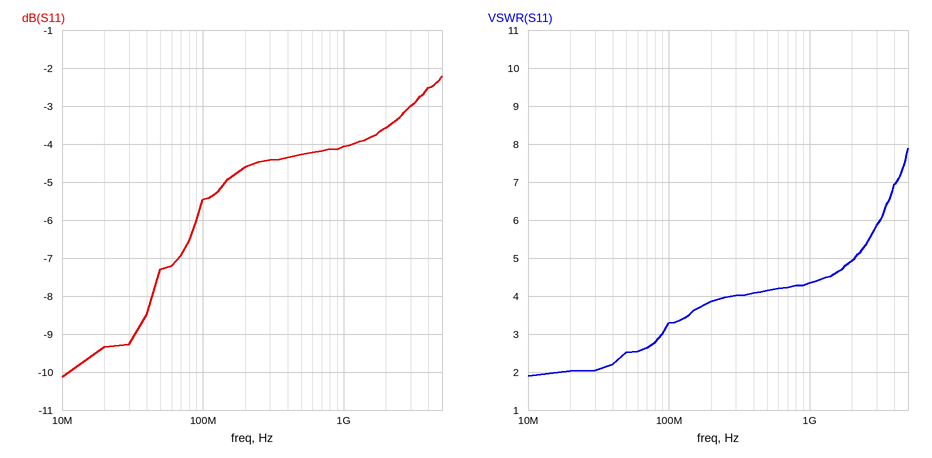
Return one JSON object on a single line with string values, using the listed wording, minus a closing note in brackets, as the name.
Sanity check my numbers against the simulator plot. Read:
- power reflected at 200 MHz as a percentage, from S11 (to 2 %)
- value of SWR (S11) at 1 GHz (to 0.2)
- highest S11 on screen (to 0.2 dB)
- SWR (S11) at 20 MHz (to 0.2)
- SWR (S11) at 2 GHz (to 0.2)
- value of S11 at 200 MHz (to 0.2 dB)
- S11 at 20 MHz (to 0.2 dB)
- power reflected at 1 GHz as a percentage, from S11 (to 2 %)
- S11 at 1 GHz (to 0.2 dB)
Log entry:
{"power reflected at 200 MHz as a percentage, from S11": "34 %", "value of SWR (S11) at 1 GHz": "4.4", "highest S11 on screen": "-2.2 dB", "SWR (S11) at 20 MHz": "2.0", "SWR (S11) at 2 GHz": "5.0", "value of S11 at 200 MHz": "-4.6 dB", "S11 at 20 MHz": "-9.4 dB", "power reflected at 1 GHz as a percentage, from S11": "40 %", "S11 at 1 GHz": "-4.0 dB"}
